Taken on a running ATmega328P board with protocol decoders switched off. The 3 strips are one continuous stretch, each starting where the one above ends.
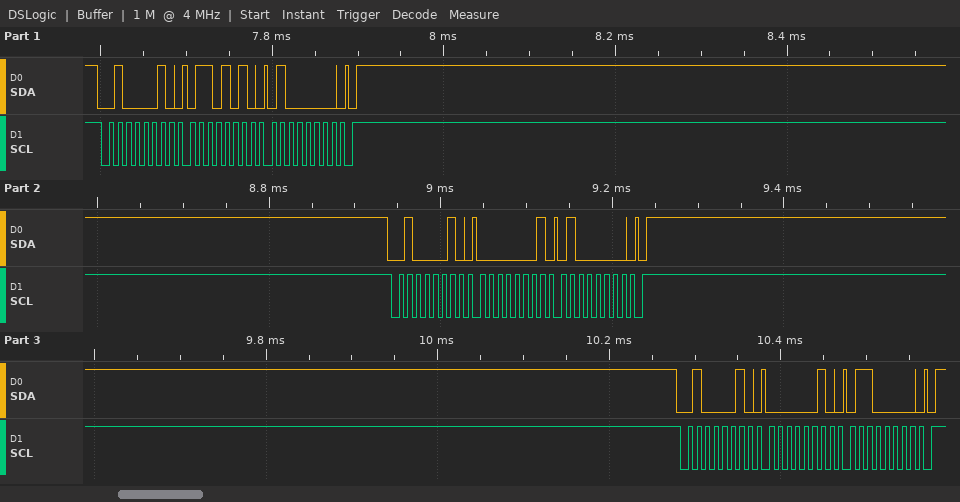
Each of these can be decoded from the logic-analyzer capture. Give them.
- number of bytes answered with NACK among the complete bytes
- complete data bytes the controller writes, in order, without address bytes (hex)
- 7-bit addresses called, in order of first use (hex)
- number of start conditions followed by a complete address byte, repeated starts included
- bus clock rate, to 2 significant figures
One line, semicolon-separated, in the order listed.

0; 6A 40 01 40 02 60; 0x21; 3; 100 kHz
